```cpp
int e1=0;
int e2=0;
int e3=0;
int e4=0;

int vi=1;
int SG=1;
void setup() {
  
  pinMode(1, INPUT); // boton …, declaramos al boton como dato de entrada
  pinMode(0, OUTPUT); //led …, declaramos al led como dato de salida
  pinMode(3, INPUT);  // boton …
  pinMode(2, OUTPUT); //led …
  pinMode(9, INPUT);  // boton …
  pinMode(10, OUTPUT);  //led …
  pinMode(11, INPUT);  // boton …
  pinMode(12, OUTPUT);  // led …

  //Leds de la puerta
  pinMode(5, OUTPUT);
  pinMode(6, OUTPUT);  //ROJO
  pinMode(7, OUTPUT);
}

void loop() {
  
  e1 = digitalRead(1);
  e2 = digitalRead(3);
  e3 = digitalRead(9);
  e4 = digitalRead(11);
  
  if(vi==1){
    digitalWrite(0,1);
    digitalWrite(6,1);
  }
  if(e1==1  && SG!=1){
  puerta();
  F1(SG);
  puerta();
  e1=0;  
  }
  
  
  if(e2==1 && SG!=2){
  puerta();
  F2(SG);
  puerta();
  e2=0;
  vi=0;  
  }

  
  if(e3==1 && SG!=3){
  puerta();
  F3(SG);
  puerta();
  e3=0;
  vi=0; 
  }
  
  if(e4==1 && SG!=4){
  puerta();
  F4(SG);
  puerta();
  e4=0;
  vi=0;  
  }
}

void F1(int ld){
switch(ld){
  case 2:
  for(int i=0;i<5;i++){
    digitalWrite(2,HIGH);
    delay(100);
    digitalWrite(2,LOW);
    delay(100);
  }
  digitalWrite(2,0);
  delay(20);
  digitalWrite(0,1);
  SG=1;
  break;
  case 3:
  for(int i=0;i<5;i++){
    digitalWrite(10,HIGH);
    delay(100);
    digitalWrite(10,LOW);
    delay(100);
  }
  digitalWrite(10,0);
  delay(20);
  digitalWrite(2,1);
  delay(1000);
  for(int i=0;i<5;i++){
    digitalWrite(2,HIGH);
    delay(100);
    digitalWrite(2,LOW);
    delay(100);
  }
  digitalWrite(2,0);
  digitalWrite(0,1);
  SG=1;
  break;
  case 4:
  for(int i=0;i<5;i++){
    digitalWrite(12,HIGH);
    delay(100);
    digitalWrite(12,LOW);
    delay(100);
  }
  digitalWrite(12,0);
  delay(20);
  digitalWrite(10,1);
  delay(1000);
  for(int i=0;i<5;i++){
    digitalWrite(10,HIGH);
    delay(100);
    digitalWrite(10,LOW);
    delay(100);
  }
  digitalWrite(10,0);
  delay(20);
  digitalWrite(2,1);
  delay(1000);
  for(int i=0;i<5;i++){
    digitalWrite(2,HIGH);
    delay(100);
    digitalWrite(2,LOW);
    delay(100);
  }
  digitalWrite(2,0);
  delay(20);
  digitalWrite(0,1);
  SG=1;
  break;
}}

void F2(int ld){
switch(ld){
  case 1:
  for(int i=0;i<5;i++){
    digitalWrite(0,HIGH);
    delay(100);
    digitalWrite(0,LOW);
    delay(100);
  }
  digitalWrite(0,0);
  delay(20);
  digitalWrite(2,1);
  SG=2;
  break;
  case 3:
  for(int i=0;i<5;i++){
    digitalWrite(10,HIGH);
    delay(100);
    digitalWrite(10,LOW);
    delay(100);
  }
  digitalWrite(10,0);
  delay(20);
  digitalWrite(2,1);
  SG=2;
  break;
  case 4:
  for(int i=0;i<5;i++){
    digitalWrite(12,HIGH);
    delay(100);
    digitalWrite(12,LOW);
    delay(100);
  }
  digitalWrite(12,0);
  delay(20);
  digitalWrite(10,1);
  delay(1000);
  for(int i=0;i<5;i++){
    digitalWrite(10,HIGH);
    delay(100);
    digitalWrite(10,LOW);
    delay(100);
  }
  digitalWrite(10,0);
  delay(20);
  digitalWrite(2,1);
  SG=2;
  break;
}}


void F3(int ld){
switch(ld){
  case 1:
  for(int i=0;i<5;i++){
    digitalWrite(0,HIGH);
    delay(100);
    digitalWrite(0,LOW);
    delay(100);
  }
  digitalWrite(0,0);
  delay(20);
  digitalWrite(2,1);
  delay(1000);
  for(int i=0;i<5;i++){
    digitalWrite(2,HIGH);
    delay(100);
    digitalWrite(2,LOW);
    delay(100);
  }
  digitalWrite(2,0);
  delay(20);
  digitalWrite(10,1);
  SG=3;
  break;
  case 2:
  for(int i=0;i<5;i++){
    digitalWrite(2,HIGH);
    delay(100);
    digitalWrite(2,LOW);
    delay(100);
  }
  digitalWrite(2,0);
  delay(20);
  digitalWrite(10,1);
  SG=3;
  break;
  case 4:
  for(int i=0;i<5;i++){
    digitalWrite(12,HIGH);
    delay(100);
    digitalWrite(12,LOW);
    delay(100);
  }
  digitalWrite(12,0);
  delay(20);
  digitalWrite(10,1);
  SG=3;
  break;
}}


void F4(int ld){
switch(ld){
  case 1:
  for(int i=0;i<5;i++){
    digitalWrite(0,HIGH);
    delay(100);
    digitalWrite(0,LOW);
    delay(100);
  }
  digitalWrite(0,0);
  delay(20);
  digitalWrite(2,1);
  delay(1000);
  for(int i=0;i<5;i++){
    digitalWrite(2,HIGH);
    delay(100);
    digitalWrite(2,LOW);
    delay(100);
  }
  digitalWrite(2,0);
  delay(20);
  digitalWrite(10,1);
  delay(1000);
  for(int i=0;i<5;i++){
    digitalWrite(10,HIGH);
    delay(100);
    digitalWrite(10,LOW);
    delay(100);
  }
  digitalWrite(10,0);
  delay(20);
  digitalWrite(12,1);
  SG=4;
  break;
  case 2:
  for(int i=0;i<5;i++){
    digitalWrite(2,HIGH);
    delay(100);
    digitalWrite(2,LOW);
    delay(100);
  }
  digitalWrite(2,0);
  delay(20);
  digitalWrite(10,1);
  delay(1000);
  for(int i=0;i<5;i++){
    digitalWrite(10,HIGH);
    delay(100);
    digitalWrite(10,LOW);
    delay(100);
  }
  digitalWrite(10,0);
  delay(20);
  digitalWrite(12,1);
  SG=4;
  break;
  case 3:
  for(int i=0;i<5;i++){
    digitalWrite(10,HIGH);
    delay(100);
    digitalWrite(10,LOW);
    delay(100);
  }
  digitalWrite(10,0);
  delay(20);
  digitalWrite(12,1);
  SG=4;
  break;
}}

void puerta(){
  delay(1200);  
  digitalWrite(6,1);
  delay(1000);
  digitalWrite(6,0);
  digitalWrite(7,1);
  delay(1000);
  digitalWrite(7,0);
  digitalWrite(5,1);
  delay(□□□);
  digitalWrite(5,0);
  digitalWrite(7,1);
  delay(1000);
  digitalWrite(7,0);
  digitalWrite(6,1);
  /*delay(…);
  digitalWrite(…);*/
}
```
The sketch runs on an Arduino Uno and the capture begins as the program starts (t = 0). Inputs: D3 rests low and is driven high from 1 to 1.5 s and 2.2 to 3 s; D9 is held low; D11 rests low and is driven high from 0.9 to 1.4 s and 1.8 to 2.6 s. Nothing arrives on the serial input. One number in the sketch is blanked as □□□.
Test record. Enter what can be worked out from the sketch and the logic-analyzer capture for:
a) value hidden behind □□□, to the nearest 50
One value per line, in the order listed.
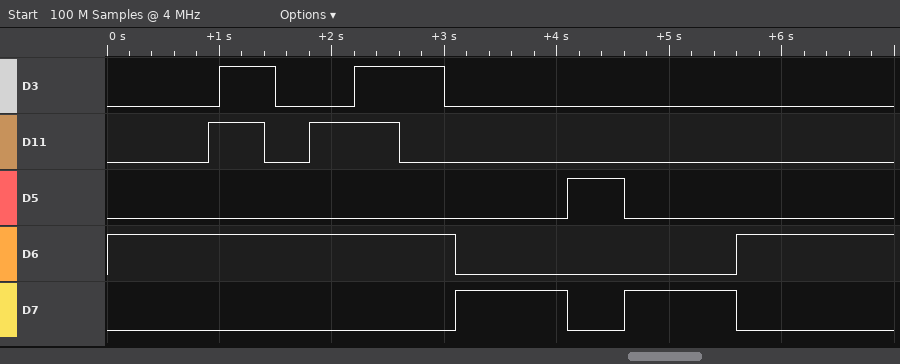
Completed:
500
